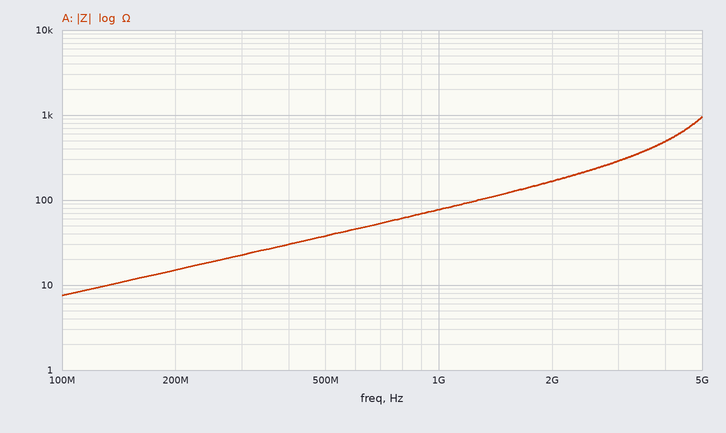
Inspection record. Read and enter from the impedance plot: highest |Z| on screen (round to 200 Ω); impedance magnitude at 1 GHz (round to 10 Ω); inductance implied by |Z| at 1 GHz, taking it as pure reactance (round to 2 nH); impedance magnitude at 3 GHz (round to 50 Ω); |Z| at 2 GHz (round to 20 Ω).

1.0 kΩ
80 Ω
12 nH
300 Ω
160 Ω
